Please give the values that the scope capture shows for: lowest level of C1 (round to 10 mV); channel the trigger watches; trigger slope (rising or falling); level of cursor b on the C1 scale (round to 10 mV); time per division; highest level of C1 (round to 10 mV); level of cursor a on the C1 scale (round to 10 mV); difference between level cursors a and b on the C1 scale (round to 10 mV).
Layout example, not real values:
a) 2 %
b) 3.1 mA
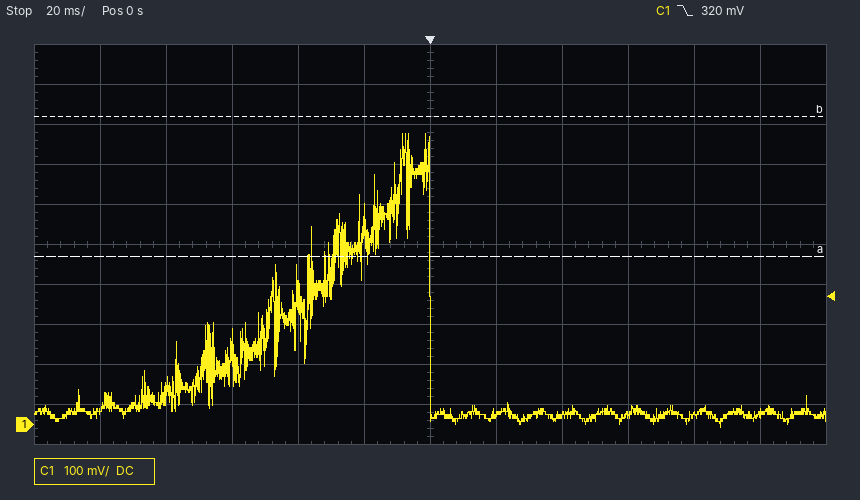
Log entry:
a) -10 mV
b) C1
c) falling
d) 770 mV
e) 20 ms
f) 730 mV
g) 420 mV
h) 350 mV
